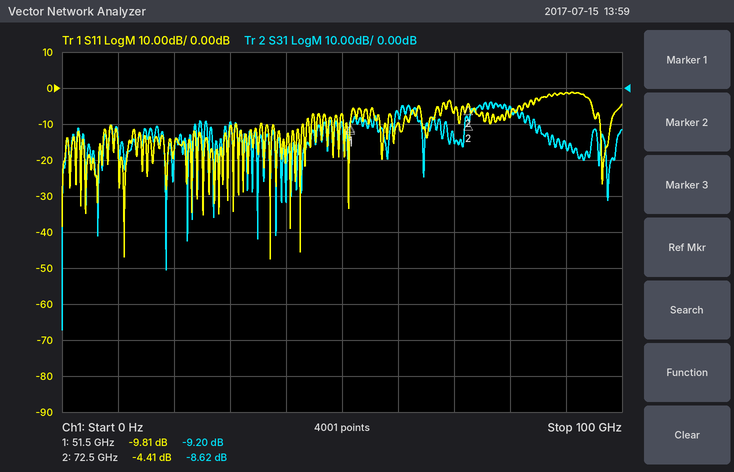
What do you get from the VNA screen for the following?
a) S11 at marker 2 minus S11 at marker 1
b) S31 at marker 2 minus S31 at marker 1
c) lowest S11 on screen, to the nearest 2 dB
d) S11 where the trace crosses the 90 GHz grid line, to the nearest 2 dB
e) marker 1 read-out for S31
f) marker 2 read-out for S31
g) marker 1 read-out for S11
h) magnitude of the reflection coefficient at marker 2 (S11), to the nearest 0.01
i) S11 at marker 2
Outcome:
5.40 dB
0.58 dB
-48 dB
-2 dB
-9.20 dB
-8.62 dB
-9.81 dB
0.60
-4.41 dB
